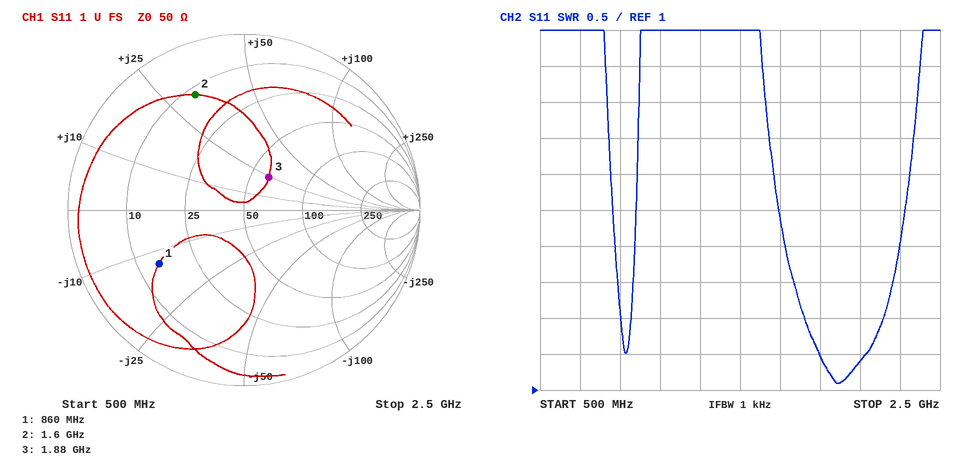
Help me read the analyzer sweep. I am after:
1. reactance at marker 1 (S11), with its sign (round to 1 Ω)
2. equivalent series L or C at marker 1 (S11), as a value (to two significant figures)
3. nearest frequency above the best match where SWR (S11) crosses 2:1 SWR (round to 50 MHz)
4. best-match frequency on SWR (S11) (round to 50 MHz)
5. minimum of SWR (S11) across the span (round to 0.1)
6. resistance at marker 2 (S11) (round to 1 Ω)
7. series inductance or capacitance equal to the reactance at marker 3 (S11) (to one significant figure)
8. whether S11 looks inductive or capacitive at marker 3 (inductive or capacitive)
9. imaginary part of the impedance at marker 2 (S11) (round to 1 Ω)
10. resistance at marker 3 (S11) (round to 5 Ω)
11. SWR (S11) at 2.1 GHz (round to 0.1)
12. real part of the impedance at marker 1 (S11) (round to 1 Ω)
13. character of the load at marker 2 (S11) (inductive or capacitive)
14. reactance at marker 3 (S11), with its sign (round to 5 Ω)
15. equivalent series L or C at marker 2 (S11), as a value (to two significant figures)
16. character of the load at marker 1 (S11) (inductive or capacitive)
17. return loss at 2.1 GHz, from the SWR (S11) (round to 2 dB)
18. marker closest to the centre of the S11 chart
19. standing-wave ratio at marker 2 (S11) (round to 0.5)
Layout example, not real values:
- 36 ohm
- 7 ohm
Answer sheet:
- -13 Ω
- 14 pF
- 2.20 GHz
- 2.00 GHz
- 1.1
- 12 Ω
- 2 nH
- inductive
- +32 Ω
- 60 Ω
- 1.4
- 15 Ω
- inductive
- +25 Ω
- 3.2 nH
- capacitive
- 16 dB
- marker 3
- 6.0
